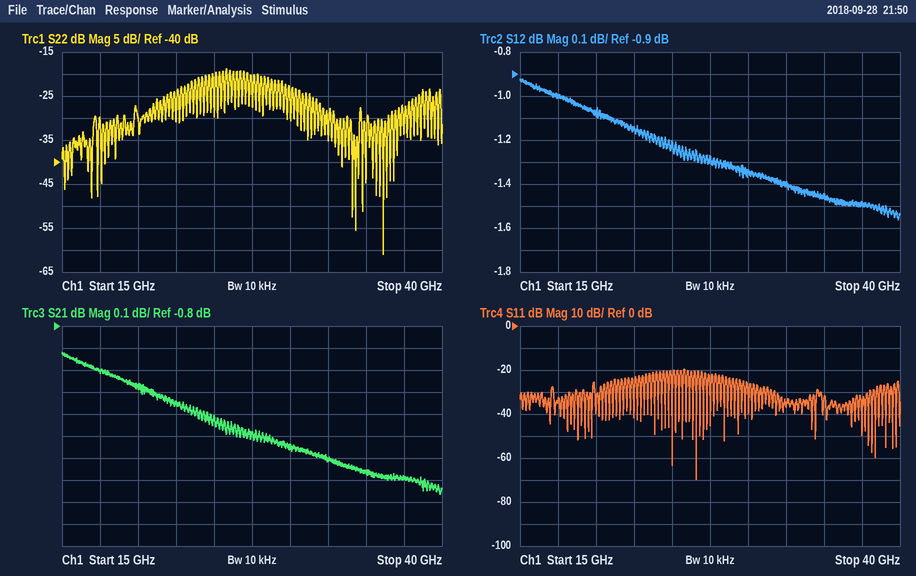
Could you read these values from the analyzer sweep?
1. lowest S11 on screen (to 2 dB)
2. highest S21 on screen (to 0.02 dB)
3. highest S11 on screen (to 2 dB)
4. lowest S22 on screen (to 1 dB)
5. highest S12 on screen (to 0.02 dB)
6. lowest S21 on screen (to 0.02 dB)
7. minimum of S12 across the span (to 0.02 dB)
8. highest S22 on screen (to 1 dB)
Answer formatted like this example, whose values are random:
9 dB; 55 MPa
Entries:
-70 dB; -0.92 dB; -20 dB; -61 dB; -0.92 dB; -1.56 dB; -1.56 dB; -19 dB
